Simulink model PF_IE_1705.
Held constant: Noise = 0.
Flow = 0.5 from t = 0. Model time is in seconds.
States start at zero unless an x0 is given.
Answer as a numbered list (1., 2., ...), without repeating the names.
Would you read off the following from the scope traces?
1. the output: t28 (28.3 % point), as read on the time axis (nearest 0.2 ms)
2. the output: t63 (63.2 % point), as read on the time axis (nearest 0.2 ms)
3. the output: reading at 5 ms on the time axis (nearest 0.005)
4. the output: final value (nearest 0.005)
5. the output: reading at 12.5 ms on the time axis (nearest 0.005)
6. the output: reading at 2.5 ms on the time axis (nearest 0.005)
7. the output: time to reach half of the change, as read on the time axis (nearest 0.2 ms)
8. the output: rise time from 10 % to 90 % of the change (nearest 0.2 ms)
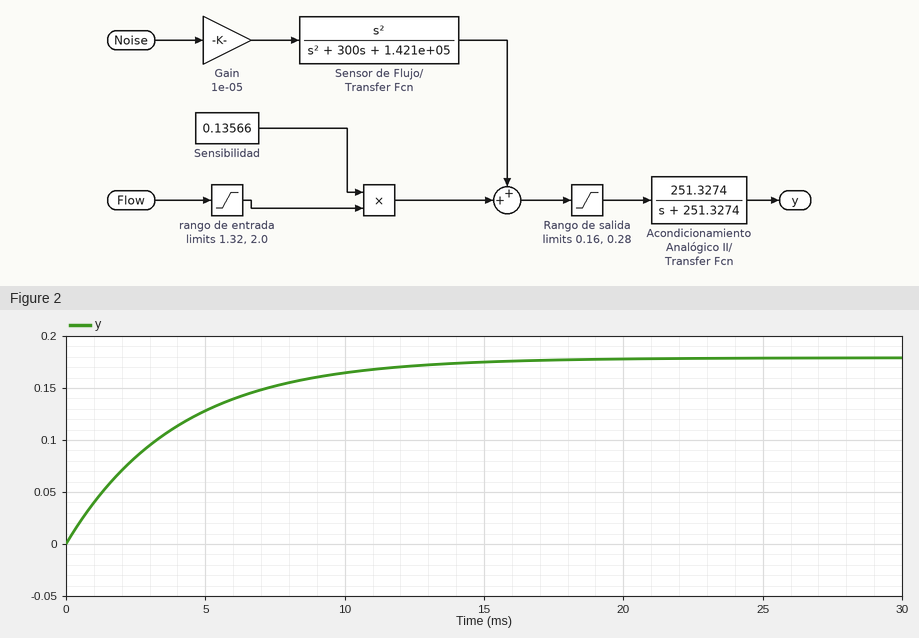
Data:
1. 1.4 ms
2. 4.0 ms
3. 0.130
4. 0.180
5. 0.170
6. 0.085
7. 2.8 ms
8. 8.8 ms
